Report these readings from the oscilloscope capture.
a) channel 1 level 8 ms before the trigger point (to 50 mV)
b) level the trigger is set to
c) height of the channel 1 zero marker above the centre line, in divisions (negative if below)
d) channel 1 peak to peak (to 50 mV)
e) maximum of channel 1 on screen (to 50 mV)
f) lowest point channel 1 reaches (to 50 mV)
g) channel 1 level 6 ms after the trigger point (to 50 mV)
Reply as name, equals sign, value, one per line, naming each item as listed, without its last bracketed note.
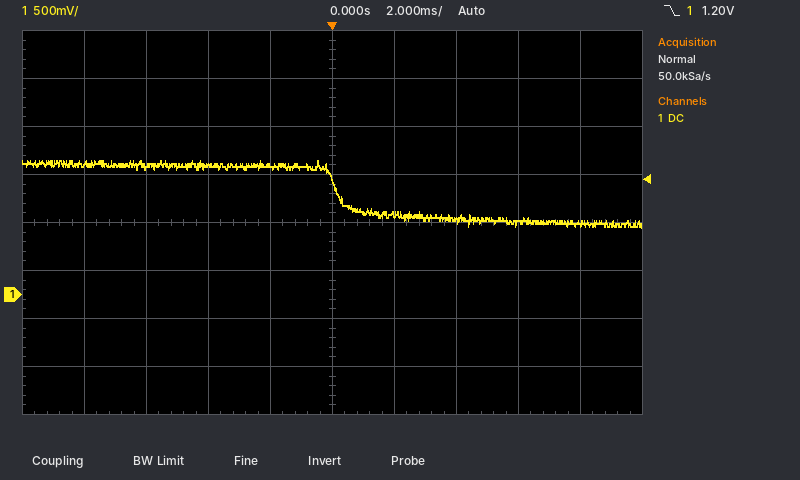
channel 1 level 8 ms before the trigger point = 1.35 V
level the trigger is set to = 1.20 V
height of the channel 1 zero marker above the centre line, in divisions = -1.5 div
channel 1 peak to peak = 700 mV
maximum of channel 1 on screen = 1.40 V
lowest point channel 1 reaches = 700 mV
channel 1 level 6 ms after the trigger point = 750 mV
